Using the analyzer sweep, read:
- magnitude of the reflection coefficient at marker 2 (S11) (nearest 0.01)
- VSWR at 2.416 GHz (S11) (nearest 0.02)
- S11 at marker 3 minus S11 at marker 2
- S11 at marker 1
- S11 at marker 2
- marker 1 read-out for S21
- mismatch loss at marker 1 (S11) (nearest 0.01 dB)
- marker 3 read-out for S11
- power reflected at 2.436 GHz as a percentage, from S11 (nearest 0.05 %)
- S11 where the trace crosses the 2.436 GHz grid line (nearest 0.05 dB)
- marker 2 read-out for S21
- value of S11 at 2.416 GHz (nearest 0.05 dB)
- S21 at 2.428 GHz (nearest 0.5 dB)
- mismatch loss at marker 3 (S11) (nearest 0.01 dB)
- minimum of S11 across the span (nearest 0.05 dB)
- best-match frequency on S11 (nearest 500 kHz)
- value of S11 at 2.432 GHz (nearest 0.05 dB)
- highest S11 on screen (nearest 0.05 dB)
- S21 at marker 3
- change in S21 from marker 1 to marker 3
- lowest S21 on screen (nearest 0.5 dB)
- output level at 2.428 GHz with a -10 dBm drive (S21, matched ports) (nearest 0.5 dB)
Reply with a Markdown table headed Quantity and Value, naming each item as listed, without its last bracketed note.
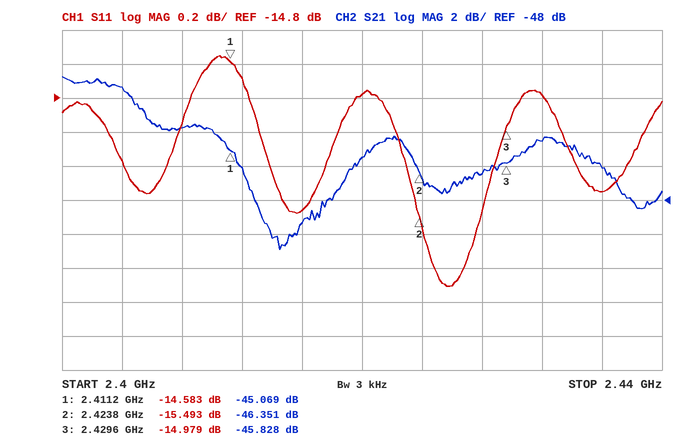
| Quantity | Value |
|---|---|
| magnitude of the reflection coefficient at marker 2 (S11) | 0.17 |
| VSWR at 2.416 GHz (S11) | 1.40 |
| S11 at marker 3 minus S11 at marker 2 | 0.514 dB |
| S11 at marker 1 | -14.583 dB |
| S11 at marker 2 | -15.493 dB |
| marker 1 read-out for S21 | -45.069 dB |
| mismatch loss at marker 1 (S11) | 0.15 dB |
| marker 3 read-out for S11 | -14.979 dB |
| power reflected at 2.436 GHz as a percentage, from S11 | 2.90 % |
| S11 where the trace crosses the 2.436 GHz grid line | -15.35 dB |
| marker 2 read-out for S21 | -46.351 dB |
| value of S11 at 2.416 GHz | -15.45 dB |
| S21 at 2.428 GHz | -46.5 dB |
| mismatch loss at marker 3 (S11) | 0.14 dB |
| minimum of S11 across the span | -15.90 dB |
| best-match frequency on S11 | 2.4255 GHz |
| value of S11 at 2.432 GHz | -14.80 dB |
| highest S11 on screen | -14.55 dB |
| S21 at marker 3 | -45.828 dB |
| change in S21 from marker 1 to marker 3 | -0.759 dB |
| lowest S21 on screen | -51.0 dB |
| output level at 2.428 GHz with a -10 dBm drive (S21, matched ports) | -56.5 dBm |
